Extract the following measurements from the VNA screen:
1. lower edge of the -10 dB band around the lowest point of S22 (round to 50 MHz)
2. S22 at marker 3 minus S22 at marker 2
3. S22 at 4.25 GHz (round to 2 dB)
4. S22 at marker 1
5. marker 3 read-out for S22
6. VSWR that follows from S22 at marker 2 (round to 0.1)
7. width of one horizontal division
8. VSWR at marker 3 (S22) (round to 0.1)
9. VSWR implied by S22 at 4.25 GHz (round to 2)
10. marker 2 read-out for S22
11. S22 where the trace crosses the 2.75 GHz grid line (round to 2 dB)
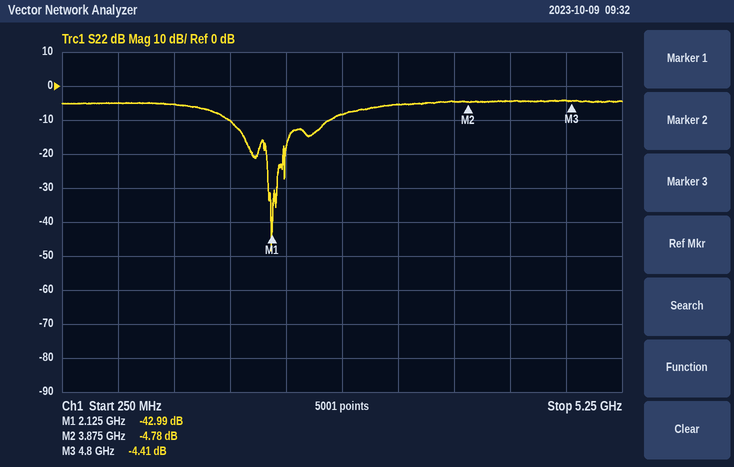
1.75 GHz
0.37 dB
-4 dB
-42.99 dB
-4.41 dB
3.7
500 MHz
4.0
4
-4.78 dB
-8 dB
